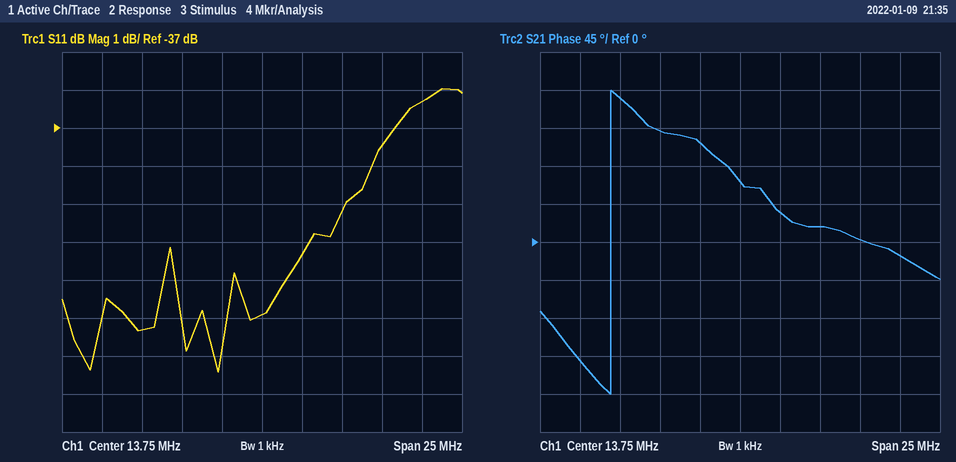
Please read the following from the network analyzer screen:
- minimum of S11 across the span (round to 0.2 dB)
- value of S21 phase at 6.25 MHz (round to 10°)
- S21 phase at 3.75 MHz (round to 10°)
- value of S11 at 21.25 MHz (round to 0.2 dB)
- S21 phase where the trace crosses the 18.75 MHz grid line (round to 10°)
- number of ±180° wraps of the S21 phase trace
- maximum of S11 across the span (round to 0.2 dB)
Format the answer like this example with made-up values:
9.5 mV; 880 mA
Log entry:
-43.4 dB; 170°; -140°; -37.4 dB; 20°; 1; -36.0 dB
